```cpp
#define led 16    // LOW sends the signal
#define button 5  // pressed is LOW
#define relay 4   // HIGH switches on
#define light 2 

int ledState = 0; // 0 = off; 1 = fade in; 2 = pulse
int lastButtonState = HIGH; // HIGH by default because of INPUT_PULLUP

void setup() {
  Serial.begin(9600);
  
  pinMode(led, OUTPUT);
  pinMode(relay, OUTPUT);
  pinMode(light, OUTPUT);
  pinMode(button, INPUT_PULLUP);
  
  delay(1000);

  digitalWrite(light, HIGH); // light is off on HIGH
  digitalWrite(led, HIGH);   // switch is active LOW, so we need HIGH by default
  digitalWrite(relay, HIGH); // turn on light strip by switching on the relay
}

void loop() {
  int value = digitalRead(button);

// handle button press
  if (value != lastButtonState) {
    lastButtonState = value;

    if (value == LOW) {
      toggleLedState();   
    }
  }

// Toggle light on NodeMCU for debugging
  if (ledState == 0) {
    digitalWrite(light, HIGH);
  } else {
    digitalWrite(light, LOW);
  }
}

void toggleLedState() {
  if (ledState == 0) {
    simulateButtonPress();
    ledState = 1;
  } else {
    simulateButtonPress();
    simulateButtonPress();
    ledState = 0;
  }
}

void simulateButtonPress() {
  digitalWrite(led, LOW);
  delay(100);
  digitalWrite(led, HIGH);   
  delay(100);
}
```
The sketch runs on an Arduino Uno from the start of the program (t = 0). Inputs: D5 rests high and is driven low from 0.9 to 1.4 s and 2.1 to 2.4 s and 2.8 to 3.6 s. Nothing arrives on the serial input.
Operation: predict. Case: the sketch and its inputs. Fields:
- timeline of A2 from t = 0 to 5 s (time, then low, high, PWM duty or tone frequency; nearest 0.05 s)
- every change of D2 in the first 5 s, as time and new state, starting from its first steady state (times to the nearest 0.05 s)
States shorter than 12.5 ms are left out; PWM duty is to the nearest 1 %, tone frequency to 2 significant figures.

0 s low; 1.1 s high; 2.1 s low; 2.2 s high; 2.3 s low; 2.4 s high; 2.8 s low; 2.9 s high
0 s low; 1 s high; 1.2 s low; 2.5 s high; 3 s low
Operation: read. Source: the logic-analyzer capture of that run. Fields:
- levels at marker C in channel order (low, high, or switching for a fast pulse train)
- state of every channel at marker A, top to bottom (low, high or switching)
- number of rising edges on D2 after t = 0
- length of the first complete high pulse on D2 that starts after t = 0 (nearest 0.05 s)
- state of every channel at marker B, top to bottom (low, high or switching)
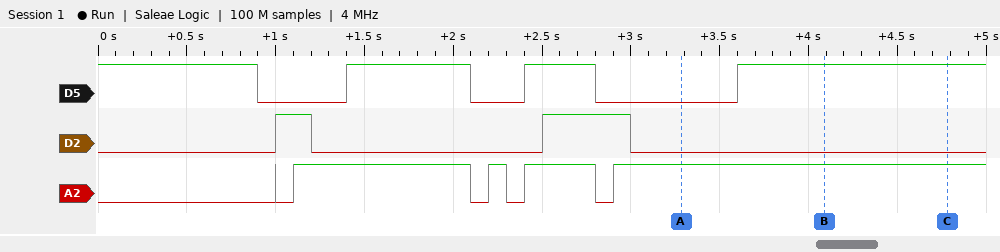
D5 high, D2 low, A2 high
D5 low, D2 low, A2 high
2
0.20 s
D5 high, D2 low, A2 high
